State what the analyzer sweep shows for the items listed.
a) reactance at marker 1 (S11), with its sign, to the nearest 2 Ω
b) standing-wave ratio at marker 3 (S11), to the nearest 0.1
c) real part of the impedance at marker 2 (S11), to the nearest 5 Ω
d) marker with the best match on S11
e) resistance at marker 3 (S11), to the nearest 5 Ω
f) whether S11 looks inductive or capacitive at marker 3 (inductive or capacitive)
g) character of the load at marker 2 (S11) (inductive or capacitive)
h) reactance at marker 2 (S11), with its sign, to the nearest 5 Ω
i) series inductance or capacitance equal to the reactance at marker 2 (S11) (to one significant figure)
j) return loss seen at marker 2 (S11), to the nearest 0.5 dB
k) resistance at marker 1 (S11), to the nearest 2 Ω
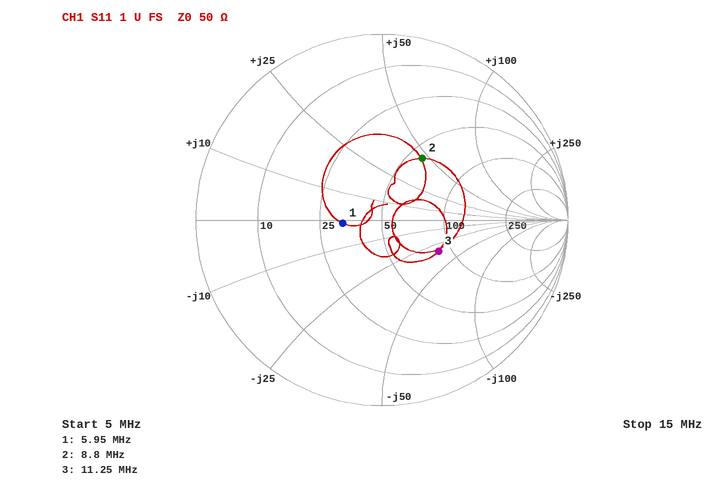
-2 Ω
2.1
60 Ω
marker 1
85 Ω
capacitive
inductive
+45 Ω
800 nH
8.0 dB
32 Ω
